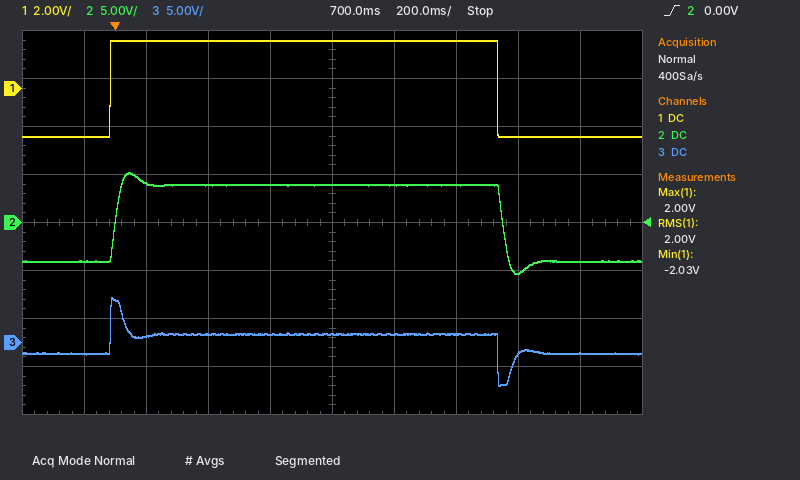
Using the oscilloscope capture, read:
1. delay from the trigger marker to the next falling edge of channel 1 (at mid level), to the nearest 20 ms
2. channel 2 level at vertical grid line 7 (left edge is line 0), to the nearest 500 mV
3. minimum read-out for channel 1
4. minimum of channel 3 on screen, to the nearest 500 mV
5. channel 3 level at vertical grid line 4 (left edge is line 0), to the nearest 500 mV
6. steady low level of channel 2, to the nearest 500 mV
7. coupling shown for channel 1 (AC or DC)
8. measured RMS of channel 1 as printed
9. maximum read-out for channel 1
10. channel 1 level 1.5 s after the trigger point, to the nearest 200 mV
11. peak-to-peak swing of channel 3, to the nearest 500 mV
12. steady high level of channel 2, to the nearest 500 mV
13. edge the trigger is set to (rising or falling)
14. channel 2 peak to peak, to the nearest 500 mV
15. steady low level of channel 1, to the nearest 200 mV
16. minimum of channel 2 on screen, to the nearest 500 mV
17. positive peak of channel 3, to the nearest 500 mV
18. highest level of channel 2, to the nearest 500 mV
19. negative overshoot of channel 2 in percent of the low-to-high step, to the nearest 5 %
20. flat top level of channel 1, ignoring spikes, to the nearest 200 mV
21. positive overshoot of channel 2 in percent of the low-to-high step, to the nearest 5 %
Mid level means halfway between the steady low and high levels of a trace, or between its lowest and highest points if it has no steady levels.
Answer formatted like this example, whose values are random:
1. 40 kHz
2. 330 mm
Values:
1. 1.24 s
2. 4.0 V
3. -2.03 V
4. -4.5 V
5. 1.0 V
6. -4.0 V
7. DC
8. 2.00 V
9. 2.00 V
10. -2.0 V
11. 9.0 V
12. 4.0 V
13. rising
14. 10.5 V
15. -2.0 V
16. -5.5 V
17. 4.5 V
18. 5.0 V
19. 15 %
20. 2.0 V
21. 15 %
